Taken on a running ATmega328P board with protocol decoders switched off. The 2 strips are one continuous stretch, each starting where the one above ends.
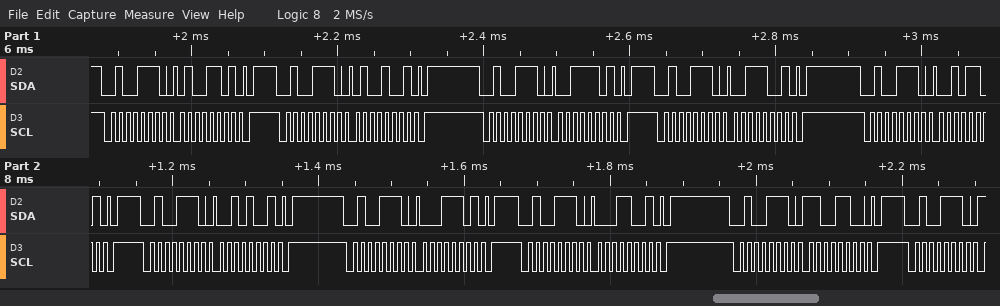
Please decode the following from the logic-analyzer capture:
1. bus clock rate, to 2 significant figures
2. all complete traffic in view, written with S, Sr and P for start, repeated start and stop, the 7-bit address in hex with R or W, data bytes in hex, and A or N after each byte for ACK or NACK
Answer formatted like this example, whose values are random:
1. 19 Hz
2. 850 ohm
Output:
1. 100 kHz
2. S 27W A 4D A P S 27W A 49 A P S 27W A 3D A P S 27W A 39 A P S 27W A 2D A P S 27W A 29 A P S 27W A 1D A P S 27W A 19 A P S 27W A CC A P S 27W A
